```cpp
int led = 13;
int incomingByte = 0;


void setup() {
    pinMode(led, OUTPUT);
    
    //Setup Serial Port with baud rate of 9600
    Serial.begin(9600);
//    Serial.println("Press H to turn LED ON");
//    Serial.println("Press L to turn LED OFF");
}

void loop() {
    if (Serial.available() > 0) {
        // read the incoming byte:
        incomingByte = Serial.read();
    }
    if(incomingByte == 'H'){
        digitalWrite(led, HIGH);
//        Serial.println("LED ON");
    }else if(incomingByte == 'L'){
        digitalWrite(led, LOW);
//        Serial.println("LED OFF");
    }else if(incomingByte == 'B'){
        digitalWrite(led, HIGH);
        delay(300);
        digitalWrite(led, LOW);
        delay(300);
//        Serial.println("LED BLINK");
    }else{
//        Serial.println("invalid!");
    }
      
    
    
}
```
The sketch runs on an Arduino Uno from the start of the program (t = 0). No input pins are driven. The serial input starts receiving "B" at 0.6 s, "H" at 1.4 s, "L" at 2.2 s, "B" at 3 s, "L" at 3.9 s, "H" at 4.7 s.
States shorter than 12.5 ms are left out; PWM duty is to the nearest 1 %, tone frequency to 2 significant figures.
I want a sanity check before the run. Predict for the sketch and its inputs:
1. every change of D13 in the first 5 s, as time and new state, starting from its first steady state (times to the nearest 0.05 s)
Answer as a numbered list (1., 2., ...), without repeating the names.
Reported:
1. 0 s low; 0.6 s high; 0.9 s low; 1.2 s high; 1.5 s low; 1.8 s high; 2.2 s low; 3 s high; 3.3 s low; 3.6 s high; 3.9 s low; 4.7 s high
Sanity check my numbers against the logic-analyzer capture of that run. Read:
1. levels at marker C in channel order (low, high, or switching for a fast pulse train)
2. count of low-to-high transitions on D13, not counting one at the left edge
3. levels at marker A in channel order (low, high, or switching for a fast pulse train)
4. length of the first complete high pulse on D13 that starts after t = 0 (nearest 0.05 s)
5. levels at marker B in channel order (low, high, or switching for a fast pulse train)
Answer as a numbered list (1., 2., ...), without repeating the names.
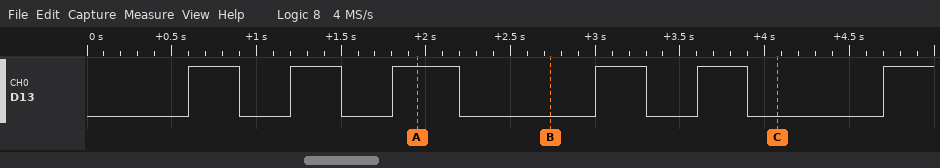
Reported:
1. D13 low
2. 6
3. D13 high
4. 0.30 s
5. D13 low
